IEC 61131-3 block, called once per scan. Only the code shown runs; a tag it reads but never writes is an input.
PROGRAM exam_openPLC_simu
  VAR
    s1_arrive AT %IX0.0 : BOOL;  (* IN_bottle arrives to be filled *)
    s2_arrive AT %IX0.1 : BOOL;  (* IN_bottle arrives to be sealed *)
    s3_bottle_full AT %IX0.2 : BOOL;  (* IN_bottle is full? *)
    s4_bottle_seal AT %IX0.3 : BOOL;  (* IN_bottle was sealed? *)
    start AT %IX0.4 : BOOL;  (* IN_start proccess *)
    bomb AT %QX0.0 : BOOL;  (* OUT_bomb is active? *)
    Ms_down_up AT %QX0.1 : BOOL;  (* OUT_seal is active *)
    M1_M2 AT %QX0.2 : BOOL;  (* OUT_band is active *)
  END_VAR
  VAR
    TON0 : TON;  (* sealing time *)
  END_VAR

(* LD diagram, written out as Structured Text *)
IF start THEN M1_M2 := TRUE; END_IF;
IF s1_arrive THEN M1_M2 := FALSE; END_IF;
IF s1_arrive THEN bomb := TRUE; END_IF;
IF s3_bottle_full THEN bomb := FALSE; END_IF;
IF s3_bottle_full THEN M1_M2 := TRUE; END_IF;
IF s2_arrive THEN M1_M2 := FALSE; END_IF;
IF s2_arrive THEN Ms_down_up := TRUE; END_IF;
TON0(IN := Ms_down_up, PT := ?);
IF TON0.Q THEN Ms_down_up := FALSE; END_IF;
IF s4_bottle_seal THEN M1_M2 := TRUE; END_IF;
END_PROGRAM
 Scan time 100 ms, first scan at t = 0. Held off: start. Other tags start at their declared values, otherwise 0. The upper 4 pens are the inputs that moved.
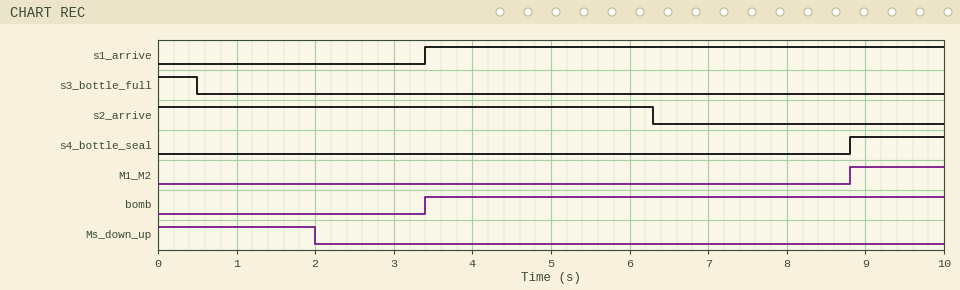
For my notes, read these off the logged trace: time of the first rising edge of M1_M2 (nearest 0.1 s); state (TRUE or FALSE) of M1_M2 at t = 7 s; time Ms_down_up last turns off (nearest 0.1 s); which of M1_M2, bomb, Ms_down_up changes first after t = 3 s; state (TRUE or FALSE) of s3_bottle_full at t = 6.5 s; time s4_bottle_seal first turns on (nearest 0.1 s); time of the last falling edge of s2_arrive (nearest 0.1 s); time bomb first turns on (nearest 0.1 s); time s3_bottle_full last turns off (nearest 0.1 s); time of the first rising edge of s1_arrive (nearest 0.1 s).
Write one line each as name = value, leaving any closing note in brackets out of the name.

time of the first rising edge of M1_M2 = 8.8 s
state (TRUE or FALSE) of M1_M2 at t = 7 s = FALSE
time Ms_down_up last turns off = 2.0 s
which of M1_M2, bomb, Ms_down_up changes first after t = 3 s = bomb
state (TRUE or FALSE) of s3_bottle_full at t = 6.5 s = FALSE
time s4_bottle_seal first turns on = 8.8 s
time of the last falling edge of s2_arrive = 6.3 s
time bomb first turns on = 3.4 s
time s3_bottle_full last turns off = 0.5 s
time of the first rising edge of s1_arrive = 3.4 s
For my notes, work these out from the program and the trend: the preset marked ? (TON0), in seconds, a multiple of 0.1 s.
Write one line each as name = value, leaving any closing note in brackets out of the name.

the preset marked ? (TON0), in seconds, a multiple of 0.1 s = 2.0 s
